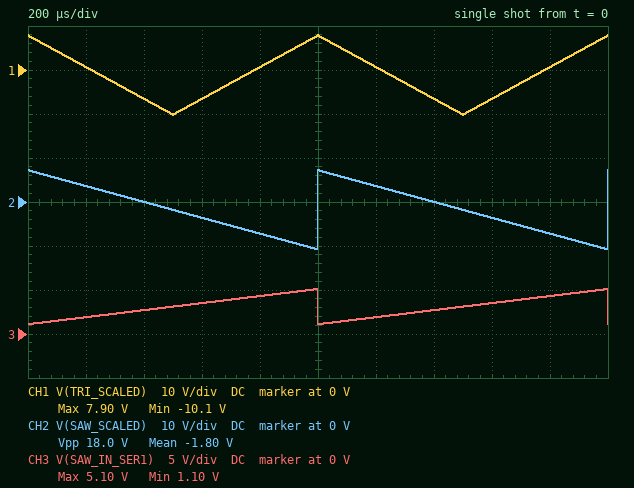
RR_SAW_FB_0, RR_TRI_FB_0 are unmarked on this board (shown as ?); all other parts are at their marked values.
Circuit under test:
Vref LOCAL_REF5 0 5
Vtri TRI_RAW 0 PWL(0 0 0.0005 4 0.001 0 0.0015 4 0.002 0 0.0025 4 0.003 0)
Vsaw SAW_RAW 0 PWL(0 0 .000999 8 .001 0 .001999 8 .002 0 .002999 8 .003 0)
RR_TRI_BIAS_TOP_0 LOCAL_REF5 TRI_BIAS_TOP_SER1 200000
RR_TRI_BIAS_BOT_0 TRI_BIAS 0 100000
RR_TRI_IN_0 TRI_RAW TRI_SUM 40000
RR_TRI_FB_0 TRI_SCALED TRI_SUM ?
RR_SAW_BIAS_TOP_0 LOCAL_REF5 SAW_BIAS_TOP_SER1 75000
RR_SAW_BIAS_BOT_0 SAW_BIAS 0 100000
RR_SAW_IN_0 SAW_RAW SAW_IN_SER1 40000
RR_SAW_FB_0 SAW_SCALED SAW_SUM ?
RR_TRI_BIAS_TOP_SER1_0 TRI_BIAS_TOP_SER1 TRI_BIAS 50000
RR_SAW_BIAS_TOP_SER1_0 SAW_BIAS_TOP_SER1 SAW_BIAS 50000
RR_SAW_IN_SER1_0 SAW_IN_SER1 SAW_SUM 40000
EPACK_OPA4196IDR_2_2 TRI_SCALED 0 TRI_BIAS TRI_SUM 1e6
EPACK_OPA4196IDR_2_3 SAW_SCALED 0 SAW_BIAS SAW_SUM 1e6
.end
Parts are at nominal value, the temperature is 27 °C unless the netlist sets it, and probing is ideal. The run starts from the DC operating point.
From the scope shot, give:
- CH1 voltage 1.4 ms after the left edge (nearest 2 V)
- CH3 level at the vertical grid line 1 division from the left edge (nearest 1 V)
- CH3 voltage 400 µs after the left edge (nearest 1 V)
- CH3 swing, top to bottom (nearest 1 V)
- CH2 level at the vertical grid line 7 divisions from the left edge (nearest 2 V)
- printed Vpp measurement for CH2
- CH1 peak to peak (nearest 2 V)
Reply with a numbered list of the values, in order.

1. -6 V
2. 2 V
3. 3 V
4. 4 V
5. 0 V
6. 18.0 V
7. 18 V
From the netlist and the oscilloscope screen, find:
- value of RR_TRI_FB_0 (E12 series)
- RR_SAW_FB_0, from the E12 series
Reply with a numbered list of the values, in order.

1. 180 kΩ
2. 180 kΩ
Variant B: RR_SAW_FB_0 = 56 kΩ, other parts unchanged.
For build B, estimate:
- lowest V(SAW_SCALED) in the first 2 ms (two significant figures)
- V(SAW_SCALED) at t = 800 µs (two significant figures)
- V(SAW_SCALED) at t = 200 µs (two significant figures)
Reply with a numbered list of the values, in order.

1. -1.8 V
2. -710 mV
3. 2.7 V
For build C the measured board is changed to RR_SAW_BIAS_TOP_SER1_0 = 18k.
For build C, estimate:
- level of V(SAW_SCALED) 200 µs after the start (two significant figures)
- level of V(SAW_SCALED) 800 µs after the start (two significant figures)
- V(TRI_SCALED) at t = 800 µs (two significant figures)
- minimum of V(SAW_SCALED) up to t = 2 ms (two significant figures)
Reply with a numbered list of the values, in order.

1. 4.8 V
2. -6.0 V
3. 660 mV
4. -9.6 V
